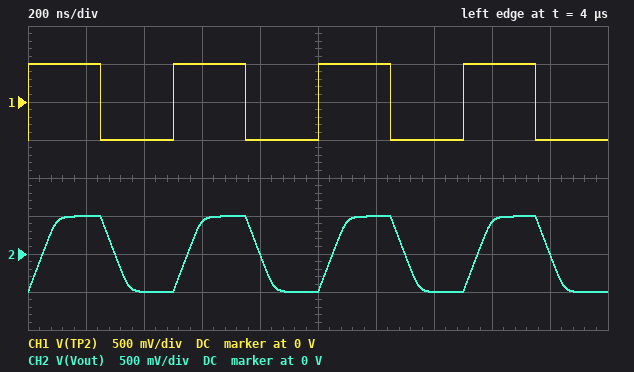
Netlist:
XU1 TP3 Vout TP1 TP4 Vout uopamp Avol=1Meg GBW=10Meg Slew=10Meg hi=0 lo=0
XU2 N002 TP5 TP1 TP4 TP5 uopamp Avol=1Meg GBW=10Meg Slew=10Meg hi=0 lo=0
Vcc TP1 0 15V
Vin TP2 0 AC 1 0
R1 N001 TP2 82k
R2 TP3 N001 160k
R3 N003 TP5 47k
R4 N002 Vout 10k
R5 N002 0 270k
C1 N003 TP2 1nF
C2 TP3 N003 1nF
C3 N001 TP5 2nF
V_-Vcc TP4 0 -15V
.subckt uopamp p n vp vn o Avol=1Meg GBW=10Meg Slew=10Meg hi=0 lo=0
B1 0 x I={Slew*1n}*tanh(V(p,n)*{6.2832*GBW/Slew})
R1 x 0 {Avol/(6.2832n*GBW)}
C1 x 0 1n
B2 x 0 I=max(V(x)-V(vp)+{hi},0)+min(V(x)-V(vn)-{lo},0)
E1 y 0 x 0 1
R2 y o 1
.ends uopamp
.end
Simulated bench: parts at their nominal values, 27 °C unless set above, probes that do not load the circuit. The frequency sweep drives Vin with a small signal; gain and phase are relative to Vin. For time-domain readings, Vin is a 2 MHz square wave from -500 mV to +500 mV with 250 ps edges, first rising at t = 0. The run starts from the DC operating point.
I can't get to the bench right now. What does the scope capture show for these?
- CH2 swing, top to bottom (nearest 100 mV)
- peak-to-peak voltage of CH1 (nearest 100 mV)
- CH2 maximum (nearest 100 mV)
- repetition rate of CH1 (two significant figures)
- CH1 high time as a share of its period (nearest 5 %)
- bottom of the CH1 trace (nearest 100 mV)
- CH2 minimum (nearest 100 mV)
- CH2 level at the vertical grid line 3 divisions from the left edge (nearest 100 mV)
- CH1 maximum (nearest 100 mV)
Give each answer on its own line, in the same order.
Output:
1.0 V
1.0 V
500 mV
2.0 MHz
50 %
-500 mV
-500 mV
400 mV
500 mV
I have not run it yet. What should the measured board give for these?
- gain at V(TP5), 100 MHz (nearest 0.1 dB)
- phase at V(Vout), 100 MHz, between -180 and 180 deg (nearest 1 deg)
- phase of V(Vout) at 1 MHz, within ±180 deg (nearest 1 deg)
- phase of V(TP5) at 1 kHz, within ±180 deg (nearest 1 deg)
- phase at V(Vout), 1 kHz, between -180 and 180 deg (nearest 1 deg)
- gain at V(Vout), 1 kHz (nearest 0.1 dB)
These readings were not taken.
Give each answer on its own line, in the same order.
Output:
-40.4 dB
-84 deg
-6 deg
-10 deg
-10 deg
0 dB
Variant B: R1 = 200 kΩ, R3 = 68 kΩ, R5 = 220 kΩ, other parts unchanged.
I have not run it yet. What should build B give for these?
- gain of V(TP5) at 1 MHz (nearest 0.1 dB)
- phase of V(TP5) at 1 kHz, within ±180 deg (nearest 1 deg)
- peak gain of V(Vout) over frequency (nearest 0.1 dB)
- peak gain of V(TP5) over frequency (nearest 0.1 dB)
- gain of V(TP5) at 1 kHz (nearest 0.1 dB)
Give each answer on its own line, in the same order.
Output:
-0.5 dB
92 deg
4.7 dB
4.3 dB
2.1 dB
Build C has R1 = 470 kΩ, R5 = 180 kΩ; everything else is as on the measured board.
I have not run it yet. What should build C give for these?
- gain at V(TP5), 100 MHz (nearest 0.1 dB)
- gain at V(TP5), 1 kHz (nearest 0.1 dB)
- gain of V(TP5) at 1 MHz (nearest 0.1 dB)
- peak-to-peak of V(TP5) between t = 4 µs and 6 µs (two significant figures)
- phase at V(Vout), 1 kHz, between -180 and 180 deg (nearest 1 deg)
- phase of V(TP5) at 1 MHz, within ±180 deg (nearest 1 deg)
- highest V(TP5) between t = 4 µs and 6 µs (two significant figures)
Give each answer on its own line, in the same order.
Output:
-40.6 dB
1.6 dB
-0.6 dB
950 mV
38 deg
-11 deg
470 mV
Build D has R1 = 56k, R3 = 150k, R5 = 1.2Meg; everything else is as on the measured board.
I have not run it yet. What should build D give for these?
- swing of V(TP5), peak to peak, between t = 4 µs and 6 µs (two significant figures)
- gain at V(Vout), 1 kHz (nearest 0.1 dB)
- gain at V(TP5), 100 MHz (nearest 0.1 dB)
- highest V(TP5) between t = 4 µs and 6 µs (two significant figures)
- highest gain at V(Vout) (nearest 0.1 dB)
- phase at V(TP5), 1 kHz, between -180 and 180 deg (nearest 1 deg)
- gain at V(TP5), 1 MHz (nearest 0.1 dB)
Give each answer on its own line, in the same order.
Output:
990 mV
-0.1 dB
-40.2 dB
490 mV
0 dB
-1 deg
-0.2 dB
